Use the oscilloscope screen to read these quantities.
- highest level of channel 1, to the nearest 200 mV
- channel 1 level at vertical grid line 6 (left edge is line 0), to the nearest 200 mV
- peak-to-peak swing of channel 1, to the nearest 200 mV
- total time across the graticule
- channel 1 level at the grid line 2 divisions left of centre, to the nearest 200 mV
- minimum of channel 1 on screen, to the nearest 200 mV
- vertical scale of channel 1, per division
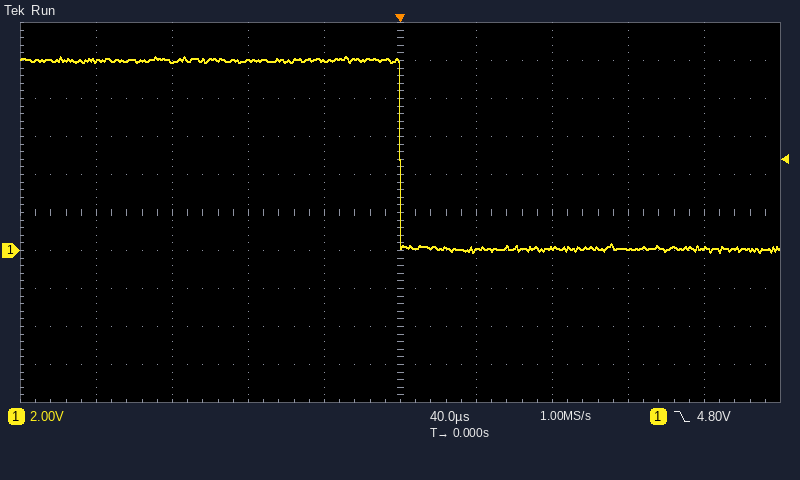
10.2 V
0.0 V
10.4 V
400 µs
10.0 V
-200 mV
2 V
